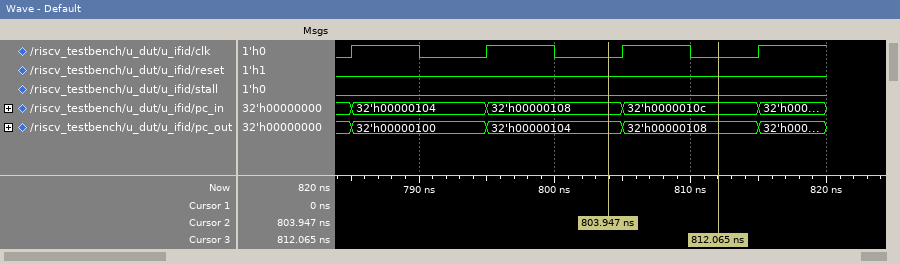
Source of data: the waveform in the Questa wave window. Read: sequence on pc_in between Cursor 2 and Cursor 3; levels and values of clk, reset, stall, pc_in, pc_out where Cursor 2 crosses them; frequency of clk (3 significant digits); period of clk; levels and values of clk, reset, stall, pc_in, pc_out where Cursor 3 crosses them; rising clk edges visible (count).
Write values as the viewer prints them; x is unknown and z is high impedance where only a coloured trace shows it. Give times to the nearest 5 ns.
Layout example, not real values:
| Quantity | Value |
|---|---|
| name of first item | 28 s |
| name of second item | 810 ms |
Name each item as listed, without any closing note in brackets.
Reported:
| Quantity | Value |
|---|---|
| sequence on pc_in between Cursor 2 and Cursor 3 | 32'h00000108, 32'h0000010c |
| levels and values of clk, reset, stall, pc_in, pc_out where Cursor 2 crosses them | clk=0, reset=0, stall=0, pc_in=32'h00000108, pc_out=32'h00000104 |
| frequency of clk | 100 MHz |
| period of clk | 10 ns |
| levels and values of clk, reset, stall, pc_in, pc_out where Cursor 3 crosses them | clk=0, reset=0, stall=0, pc_in=32'h0000010c, pc_out=32'h00000108 |
| rising clk edges visible | 4 |
